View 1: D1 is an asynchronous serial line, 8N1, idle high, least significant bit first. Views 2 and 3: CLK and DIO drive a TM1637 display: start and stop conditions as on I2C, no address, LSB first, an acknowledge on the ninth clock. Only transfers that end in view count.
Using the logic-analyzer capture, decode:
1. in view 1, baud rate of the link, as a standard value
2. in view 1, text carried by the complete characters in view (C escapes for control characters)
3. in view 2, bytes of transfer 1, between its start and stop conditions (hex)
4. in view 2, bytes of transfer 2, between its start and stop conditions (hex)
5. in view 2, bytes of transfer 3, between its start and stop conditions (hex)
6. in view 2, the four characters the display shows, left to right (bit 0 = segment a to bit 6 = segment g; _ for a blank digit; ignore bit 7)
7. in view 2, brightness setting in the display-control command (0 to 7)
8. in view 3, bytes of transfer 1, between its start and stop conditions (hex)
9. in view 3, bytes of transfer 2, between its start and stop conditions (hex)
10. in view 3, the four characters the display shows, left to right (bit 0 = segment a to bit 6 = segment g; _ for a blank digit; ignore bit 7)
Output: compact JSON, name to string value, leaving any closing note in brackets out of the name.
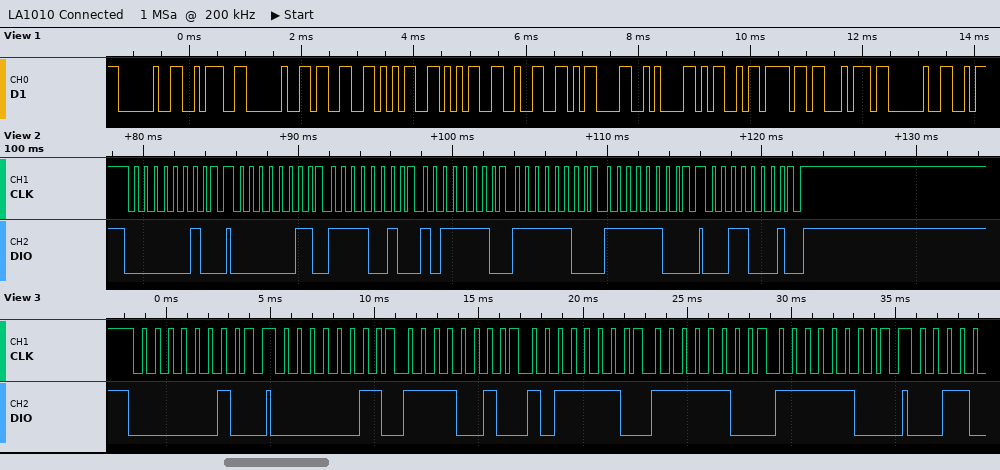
{"in view 1, baud rate of the link, as a standard value": "9600 baud", "in view 1, text carried by the complete characters in view": "\" : 3552\\r\\nMot \"", "in view 2, bytes of transfer 1, between its start and stop conditions": "40", "in view 2, bytes of transfer 2, between its start and stop conditions": "C0 4F 7D 3F 3F", "in view 2, bytes of transfer 3, between its start and stop conditions": "8C", "in view 2, the four characters the display shows, left to right": "3600", "in view 2, brightness setting in the display-control command": "4", "in view 3, bytes of transfer 1, between its start and stop conditions": "40", "in view 3, bytes of transfer 2, between its start and stop conditions": "C0 4F 7D 3F 3F", "in view 3, the four characters the display shows, left to right": "3600"}
